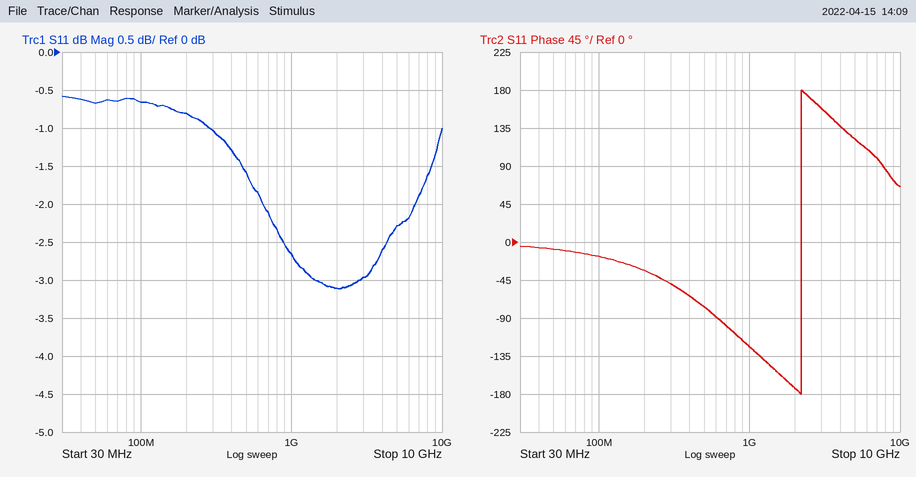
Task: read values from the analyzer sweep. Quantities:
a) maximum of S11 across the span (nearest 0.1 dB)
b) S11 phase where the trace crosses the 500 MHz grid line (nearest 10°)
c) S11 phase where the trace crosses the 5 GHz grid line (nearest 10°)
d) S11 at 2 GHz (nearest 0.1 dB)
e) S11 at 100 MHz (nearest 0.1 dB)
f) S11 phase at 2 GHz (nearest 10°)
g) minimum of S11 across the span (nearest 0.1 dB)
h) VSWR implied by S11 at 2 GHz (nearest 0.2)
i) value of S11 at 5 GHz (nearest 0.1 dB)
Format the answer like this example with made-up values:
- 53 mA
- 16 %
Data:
- -0.6 dB
- -80°
- 120°
- -3.1 dB
- -0.7 dB
- -170°
- -3.1 dB
- 5.6
- -2.3 dB
